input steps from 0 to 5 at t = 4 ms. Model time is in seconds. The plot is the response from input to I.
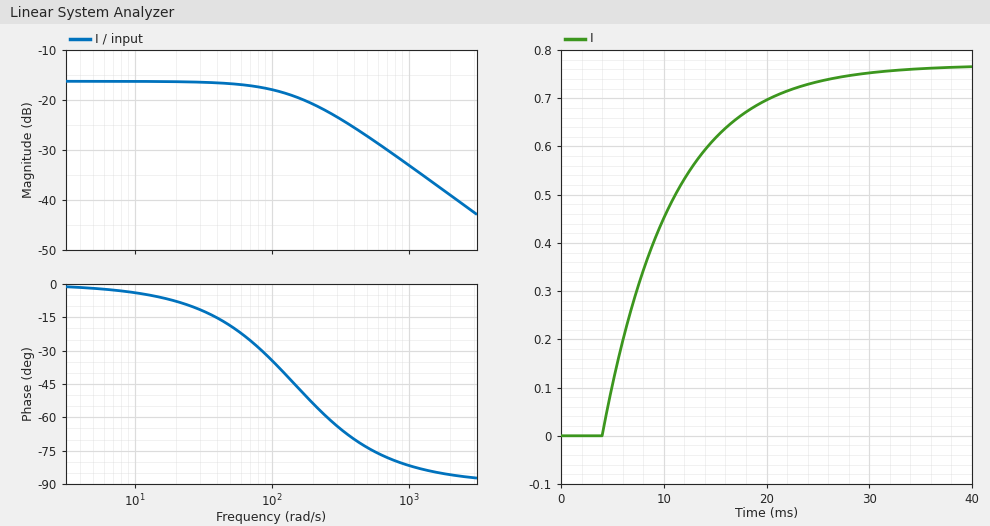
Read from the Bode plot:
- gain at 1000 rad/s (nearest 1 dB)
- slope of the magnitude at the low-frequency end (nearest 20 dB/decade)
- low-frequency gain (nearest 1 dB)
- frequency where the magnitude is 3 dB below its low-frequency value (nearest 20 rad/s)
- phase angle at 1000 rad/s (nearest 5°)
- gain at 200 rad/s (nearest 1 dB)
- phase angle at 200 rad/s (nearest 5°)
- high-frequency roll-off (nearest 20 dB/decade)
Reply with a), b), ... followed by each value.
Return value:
a) -33 dB
b) 0 dB/decade
c) -16 dB
d) 140 rad/s
e) -80°
f) -21 dB
g) -55°
h) -20 dB/decade
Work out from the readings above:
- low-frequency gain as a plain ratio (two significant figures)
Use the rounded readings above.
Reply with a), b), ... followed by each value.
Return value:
a) 0.16
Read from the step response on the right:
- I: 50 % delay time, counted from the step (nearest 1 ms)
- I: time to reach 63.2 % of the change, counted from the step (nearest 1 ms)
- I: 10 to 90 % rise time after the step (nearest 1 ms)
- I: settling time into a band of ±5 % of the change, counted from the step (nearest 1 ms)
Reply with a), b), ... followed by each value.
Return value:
a) 5 ms
b) 7 ms
c) 15 ms
d) 20 ms
